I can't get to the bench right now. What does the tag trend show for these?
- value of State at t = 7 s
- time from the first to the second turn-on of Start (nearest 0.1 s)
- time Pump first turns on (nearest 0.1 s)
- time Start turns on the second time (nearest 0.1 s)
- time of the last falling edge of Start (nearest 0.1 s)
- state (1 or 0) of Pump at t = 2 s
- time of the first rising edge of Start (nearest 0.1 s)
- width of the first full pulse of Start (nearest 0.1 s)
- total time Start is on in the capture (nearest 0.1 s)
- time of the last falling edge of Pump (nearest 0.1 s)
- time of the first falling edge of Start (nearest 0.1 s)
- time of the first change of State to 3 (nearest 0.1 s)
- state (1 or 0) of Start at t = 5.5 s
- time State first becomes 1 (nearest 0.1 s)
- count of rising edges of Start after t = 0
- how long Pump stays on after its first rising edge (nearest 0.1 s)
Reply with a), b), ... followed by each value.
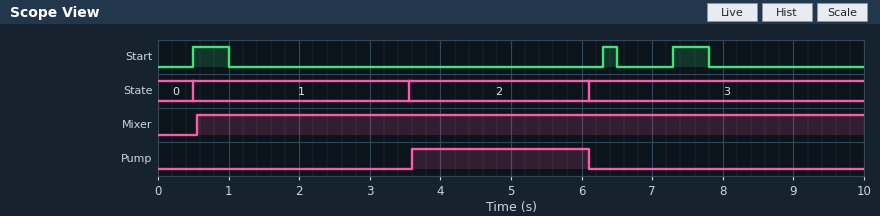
a) 3
b) 5.8 s
c) 3.6 s
d) 6.3 s
e) 7.8 s
f) 0
g) 0.5 s
h) 0.5 s
i) 1.2 s
j) 6.1 s
k) 1.0 s
l) 6.1 s
m) 0
n) 0.5 s
o) 3
p) 2.5 s
